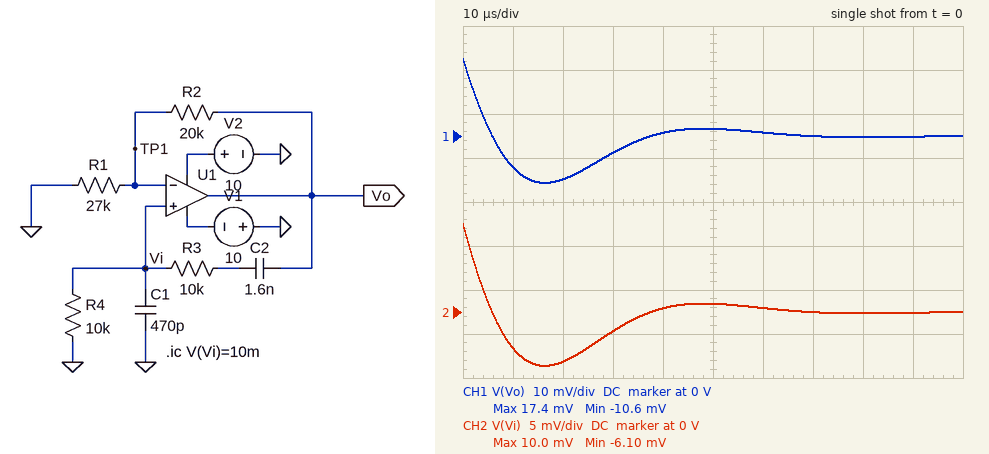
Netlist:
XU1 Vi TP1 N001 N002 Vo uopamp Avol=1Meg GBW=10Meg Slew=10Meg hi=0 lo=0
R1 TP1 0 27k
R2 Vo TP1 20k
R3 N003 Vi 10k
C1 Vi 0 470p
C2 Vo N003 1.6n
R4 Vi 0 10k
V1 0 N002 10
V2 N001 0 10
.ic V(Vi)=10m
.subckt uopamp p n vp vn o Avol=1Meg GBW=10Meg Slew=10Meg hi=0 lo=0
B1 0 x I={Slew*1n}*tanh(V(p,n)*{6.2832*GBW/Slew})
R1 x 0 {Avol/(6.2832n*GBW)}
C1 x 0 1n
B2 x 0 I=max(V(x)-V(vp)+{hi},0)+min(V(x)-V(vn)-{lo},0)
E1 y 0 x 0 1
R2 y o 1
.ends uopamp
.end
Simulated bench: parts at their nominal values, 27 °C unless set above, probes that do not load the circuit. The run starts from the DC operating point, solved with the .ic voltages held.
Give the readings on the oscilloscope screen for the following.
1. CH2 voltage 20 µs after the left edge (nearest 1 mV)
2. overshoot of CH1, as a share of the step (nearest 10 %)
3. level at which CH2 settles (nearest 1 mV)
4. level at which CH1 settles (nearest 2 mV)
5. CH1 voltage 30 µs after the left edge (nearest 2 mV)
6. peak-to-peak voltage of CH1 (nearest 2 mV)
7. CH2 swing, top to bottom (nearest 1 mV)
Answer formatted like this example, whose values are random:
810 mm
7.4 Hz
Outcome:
-6 mV
60 %
0 V
0 V
-4 mV
28 mV
16 mV
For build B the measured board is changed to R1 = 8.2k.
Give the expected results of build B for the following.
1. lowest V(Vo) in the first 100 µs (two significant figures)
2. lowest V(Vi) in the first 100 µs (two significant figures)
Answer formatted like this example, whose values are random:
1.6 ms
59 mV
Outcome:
-10 V
-5.6 V
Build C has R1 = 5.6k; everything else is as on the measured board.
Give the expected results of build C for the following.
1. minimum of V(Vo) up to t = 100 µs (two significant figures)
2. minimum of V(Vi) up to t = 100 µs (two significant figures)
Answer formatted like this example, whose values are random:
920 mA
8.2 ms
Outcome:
-10 V
-5.8 V
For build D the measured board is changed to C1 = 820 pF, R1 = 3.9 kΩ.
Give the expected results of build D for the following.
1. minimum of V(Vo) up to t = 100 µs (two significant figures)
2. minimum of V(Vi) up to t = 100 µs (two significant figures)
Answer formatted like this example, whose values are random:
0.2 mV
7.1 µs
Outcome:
-10 V
-3.4 V
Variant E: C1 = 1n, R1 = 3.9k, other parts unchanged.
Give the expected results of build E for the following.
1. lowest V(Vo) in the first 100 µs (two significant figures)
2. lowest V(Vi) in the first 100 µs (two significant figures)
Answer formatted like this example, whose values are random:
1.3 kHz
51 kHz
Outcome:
-10 V
-3.2 V
